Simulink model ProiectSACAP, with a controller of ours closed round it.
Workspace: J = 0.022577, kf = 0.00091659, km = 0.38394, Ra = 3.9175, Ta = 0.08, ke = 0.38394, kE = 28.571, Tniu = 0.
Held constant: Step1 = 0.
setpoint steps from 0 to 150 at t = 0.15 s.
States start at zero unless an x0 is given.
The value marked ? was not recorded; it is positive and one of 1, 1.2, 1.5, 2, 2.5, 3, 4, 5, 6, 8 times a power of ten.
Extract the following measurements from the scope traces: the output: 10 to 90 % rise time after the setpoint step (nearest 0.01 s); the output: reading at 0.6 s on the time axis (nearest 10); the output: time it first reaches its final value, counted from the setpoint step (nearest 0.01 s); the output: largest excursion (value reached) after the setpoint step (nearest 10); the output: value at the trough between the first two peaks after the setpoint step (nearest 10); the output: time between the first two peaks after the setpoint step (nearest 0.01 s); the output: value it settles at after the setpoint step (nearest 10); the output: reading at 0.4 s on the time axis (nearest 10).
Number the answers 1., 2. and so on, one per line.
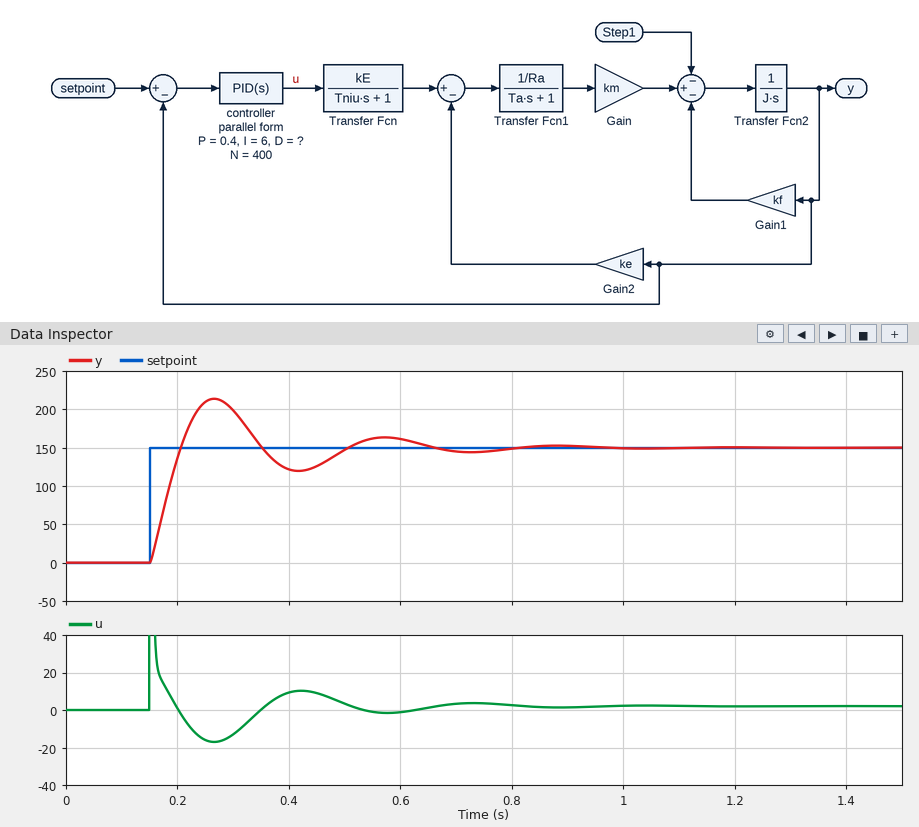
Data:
1. 0.04 s
2. 160
3. 0.06 s
4. 210
5. 120
6. 0.31 s
7. 150
8. 120
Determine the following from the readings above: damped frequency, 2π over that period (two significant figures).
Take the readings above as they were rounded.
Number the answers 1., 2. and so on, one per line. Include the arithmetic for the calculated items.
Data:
1. 2π / 0.31 = 20 rad/s
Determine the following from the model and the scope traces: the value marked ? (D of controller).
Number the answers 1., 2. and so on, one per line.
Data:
1. 0.012
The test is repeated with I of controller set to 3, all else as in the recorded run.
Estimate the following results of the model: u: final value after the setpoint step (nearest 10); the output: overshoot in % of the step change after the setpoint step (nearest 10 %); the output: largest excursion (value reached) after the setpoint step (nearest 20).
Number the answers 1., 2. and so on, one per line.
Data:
1. 0
2. 30 %
3. 200
